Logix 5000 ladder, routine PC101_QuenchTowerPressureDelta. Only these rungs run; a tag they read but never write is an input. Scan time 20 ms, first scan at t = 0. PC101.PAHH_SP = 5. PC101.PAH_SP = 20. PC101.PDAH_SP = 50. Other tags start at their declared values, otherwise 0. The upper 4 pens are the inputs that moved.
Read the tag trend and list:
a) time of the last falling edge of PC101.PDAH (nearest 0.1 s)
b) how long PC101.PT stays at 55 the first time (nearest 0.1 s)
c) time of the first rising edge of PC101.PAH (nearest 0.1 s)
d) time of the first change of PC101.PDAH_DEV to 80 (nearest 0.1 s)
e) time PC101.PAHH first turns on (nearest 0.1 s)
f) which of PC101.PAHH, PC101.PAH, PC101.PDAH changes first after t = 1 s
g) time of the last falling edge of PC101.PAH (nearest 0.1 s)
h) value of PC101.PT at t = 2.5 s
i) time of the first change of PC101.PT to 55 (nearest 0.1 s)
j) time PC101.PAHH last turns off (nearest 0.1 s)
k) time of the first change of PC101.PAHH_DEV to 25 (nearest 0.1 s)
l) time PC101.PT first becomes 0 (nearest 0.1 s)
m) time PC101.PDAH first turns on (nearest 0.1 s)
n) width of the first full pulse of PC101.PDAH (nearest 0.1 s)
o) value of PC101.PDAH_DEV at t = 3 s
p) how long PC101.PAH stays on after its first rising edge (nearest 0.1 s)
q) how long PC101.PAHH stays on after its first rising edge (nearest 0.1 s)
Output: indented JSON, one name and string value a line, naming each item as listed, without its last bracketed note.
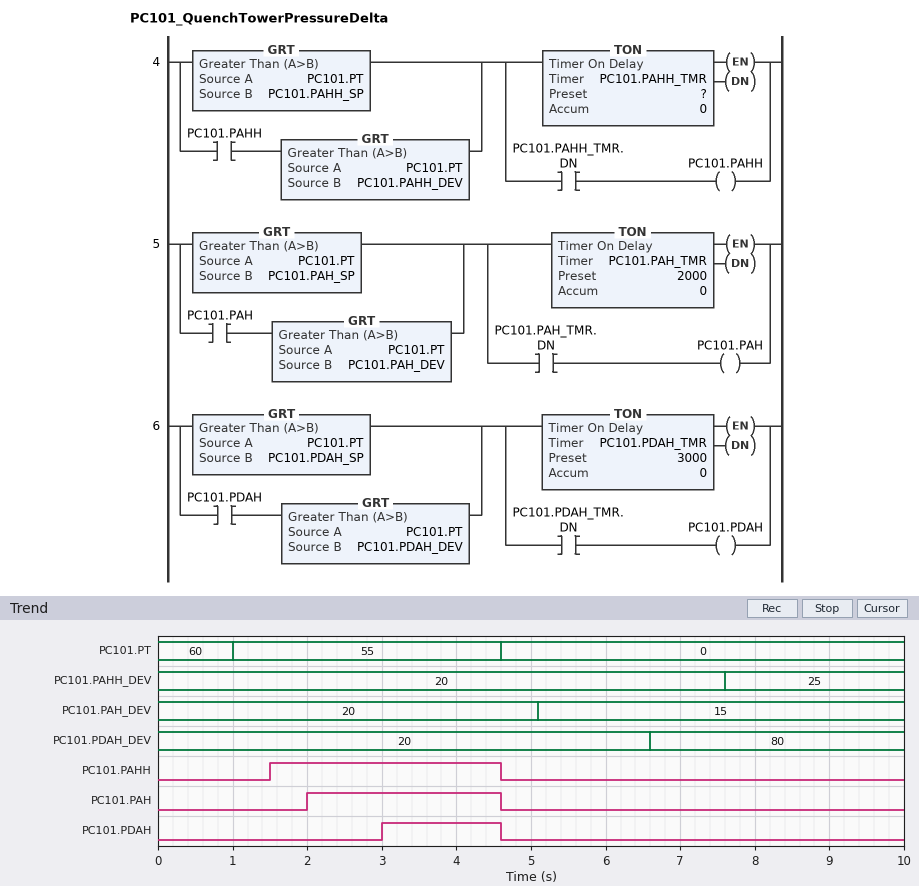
{
  "time of the last falling edge of PC101.PDAH": "4.6 s",
  "how long PC101.PT stays at 55 the first time": "3.6 s",
  "time of the first rising edge of PC101.PAH": "2.0 s",
  "time of the first change of PC101.PDAH_DEV to 80": "6.6 s",
  "time PC101.PAHH first turns on": "1.5 s",
  "which of PC101.PAHH, PC101.PAH, PC101.PDAH changes first after t = 1 s": "PC101.PAHH",
  "time of the last falling edge of PC101.PAH": "4.6 s",
  "value of PC101.PT at t = 2.5 s": "55",
  "time of the first change of PC101.PT to 55": "1.0 s",
  "time PC101.PAHH last turns off": "4.6 s",
  "time of the first change of PC101.PAHH_DEV to 25": "7.6 s",
  "time PC101.PT first becomes 0": "4.6 s",
  "time PC101.PDAH first turns on": "3.0 s",
  "width of the first full pulse of PC101.PDAH": "1.6 s",
  "value of PC101.PDAH_DEV at t = 3 s": "20",
  "how long PC101.PAH stays on after its first rising edge": "2.6 s",
  "how long PC101.PAHH stays on after its first rising edge": "3.1 s"
}
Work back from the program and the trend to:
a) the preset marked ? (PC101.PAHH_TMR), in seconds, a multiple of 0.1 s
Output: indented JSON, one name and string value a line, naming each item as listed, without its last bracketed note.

{
  "the preset marked ? (PC101.PAHH_TMR), in seconds, a multiple of 0.1 s": "1.5 s"
}
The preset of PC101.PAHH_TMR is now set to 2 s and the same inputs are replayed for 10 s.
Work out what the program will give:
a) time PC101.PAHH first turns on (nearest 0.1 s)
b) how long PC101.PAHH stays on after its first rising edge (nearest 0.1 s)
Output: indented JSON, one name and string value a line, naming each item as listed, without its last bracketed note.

{
  "time PC101.PAHH first turns on": "2.0 s",
  "how long PC101.PAHH stays on after its first rising edge": "2.6 s"
}
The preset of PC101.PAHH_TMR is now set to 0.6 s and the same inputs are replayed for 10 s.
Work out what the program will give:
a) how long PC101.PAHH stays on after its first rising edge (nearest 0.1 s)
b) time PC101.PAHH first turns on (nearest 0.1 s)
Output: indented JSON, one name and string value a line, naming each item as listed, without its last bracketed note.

{
  "how long PC101.PAHH stays on after its first rising edge": "4.0 s",
  "time PC101.PAHH first turns on": "0.6 s"
}
